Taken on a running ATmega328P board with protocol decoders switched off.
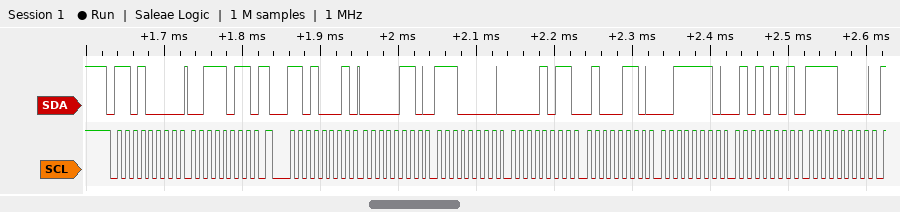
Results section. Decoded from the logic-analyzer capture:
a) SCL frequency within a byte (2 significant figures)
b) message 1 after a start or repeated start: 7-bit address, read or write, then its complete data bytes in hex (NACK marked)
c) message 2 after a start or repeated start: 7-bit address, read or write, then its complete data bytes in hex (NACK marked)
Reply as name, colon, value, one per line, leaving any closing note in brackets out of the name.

SCL frequency within a byte: 100 kHz
message 1 after a start or repeated start: 7-bit address, read or write, then its complete data bytes in hex: 0x68 write: 3B
message 2 after a start or repeated start: 7-bit address, read or write, then its complete data bytes in hex: 0x68 read: 06 E0 0B 46 3E 55 F0
